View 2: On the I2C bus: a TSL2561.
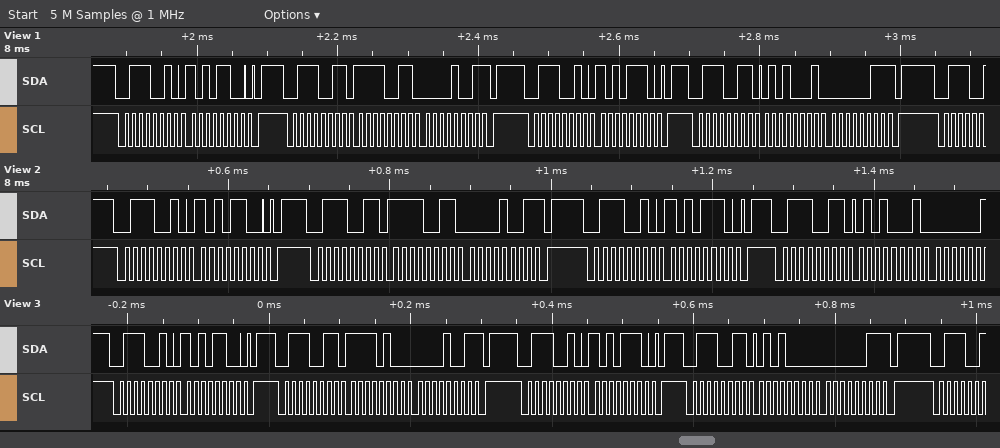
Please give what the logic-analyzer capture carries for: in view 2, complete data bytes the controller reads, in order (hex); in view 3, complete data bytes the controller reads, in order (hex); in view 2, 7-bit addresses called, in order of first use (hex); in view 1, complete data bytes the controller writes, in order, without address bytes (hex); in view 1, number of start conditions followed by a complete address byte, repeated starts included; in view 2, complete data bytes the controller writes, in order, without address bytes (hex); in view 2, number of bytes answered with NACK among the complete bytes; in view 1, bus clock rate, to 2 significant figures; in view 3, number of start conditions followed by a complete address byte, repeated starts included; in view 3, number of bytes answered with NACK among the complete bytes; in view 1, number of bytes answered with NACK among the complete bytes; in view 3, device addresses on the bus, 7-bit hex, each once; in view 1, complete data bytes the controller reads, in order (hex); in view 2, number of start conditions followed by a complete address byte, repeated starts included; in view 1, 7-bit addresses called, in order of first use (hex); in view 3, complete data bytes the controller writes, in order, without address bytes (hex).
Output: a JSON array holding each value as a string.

["F3 09 51", "F4 09 50 03", "0x39", "AC AE", "4", "AC AE", "1", "100 kHz", "4", "2", "2", "0x39", "F3 09 51 03", "4", "0x39", "AC AE"]
